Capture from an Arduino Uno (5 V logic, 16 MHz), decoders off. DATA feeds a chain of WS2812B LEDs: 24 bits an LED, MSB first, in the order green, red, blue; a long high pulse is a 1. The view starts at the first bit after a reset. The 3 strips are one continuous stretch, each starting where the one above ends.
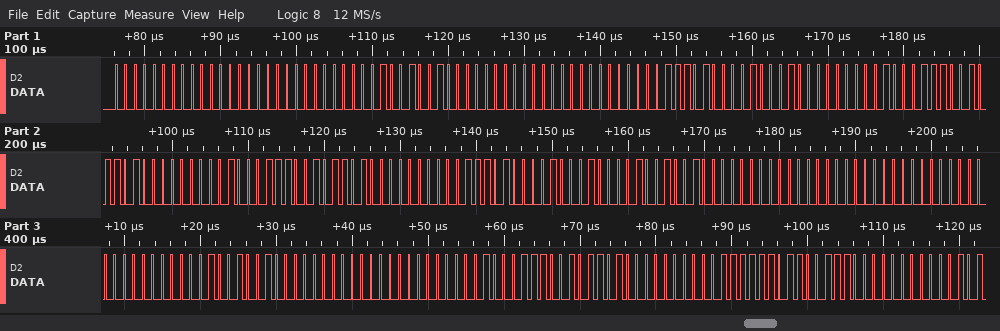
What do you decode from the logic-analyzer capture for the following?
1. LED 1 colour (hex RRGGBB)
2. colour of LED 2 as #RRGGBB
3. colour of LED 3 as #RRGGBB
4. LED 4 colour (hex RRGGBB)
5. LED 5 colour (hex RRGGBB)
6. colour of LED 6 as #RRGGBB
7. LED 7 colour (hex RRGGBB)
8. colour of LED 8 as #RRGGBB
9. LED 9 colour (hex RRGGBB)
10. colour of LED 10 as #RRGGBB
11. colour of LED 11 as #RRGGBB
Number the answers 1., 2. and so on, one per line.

1. #000000
2. #200900
3. #3A0011
4. #47002D
5. #47002D
6. #3A0011
7. #200900
8. #000000
9. #200900
10. #47002D
11. #3F0067
